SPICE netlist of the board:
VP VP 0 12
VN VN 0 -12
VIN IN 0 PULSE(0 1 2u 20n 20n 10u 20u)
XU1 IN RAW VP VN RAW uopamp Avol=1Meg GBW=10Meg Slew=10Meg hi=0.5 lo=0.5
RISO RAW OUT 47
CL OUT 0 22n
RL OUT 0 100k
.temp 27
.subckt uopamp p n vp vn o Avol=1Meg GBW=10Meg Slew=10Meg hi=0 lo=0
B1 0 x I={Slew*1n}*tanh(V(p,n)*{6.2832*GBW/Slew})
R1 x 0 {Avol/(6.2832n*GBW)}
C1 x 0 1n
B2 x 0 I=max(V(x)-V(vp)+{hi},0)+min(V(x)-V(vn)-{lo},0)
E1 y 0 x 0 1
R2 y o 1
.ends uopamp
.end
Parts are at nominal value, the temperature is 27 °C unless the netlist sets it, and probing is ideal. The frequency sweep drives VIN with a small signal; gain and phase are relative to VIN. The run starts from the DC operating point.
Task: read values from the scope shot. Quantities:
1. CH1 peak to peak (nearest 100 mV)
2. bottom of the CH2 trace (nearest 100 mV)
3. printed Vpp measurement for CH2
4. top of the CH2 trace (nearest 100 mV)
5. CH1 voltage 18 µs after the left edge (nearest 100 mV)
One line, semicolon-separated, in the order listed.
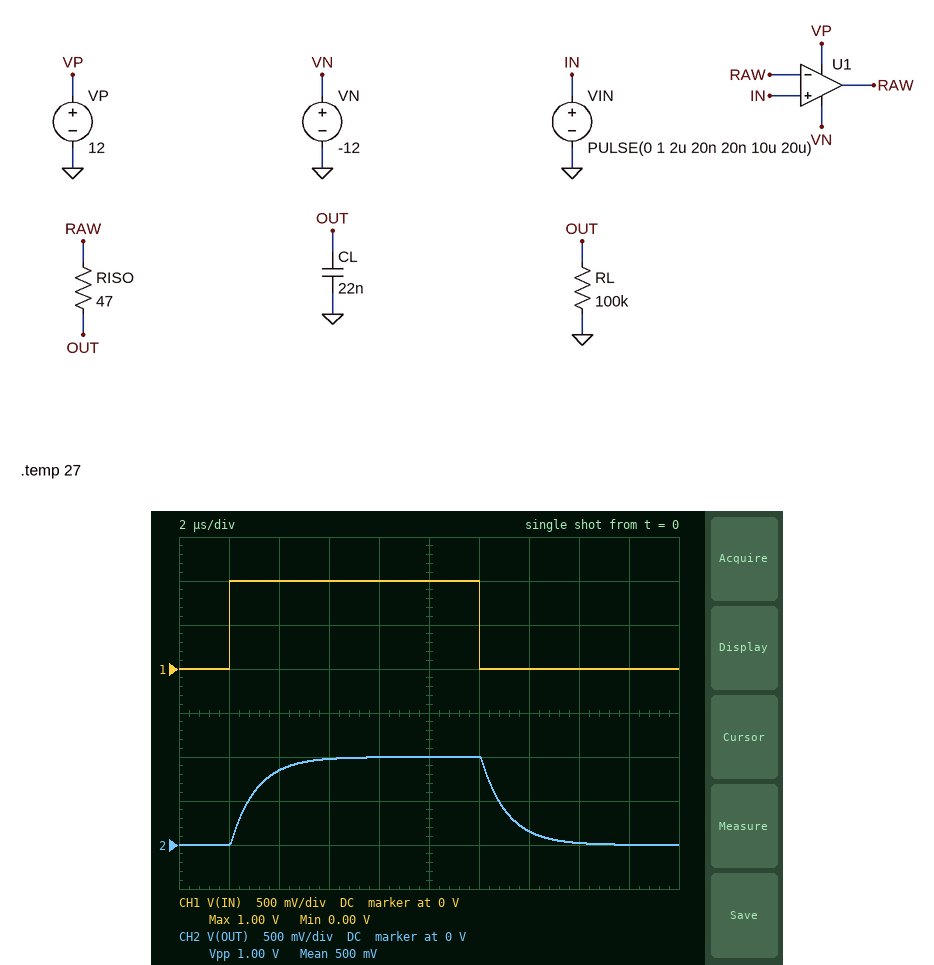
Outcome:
1.0 V; 0 V; 1.00 V; 1.0 V; 0 V
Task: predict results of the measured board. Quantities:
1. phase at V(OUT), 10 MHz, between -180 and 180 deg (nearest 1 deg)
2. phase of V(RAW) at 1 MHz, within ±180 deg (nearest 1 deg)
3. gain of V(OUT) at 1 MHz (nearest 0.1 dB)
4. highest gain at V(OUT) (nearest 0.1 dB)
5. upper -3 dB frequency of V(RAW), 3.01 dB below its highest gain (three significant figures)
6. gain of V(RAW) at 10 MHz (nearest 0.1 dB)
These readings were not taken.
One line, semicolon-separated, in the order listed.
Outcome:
-135 deg; -6 deg; -16.4 dB; 0 dB; 9.79 MHz; -3.1 dB
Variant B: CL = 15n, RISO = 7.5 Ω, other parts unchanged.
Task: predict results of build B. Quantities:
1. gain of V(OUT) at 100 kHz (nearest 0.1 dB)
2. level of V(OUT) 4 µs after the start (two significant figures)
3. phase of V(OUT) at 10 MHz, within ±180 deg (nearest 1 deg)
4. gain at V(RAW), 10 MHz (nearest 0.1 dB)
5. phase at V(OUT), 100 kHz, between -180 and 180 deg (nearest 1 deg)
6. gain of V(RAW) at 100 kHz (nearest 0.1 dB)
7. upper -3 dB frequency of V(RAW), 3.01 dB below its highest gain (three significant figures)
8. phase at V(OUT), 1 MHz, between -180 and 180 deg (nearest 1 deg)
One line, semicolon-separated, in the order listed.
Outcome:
0 dB; 1.0 V; -131 deg; -3.5 dB; -5 deg; 0 dB; 8.99 MHz; -41 deg
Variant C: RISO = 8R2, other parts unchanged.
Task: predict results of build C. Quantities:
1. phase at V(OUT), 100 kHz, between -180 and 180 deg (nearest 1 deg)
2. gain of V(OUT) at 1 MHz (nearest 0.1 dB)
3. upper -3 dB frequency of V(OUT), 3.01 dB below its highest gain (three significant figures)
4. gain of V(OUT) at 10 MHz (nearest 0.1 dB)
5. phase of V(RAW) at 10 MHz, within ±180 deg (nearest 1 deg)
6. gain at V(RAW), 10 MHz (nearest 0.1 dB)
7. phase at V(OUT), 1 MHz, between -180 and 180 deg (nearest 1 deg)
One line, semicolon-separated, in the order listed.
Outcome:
-7 deg; -3.6 dB; 884 kHz; -24.6 dB; -49 deg; -3.5 dB; -55 deg
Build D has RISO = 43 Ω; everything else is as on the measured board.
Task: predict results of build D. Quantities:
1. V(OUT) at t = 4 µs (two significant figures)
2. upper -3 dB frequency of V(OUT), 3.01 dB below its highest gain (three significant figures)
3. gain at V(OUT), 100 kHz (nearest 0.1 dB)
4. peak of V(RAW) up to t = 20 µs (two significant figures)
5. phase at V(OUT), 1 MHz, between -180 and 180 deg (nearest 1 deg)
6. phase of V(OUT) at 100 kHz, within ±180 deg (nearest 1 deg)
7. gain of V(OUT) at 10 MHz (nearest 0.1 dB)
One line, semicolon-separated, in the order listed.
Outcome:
870 mV; 168 kHz; -1.3 dB; 1.0 V; -86 deg; -31 deg; -38.6 dB
